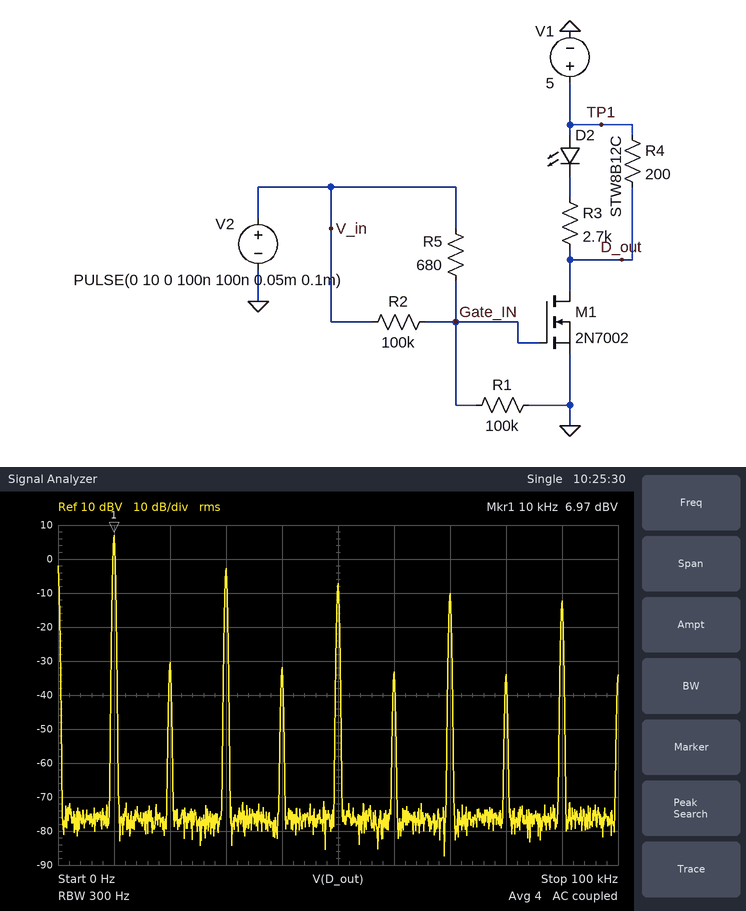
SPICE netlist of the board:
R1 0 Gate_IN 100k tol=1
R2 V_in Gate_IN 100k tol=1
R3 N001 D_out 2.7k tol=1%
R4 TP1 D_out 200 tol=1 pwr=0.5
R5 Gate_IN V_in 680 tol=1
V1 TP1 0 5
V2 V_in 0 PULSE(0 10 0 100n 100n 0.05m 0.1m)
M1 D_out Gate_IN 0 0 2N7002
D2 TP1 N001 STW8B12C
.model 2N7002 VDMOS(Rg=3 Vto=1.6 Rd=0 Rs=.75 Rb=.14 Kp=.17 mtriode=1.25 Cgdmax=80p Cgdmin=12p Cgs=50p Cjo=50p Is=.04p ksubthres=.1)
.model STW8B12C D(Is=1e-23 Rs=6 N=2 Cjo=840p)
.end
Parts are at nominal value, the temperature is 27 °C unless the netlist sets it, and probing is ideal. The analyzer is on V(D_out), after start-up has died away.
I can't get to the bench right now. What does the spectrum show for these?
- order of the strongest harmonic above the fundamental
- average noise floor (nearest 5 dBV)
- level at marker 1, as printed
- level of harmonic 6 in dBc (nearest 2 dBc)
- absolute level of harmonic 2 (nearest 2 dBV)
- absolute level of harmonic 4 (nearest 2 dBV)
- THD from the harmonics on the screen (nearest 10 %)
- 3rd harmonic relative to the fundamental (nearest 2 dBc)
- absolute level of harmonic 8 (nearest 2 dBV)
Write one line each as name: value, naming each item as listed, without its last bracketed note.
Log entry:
order of the strongest harmonic above the fundamental: 3
average noise floor: -75 dBV
level at marker 1, as printed: 6.97 dBV
level of harmonic 6 in dBc: -40 dBc
absolute level of harmonic 2: -30 dBV
absolute level of harmonic 4: -32 dBV
THD from the harmonics on the screen: 40 %
3rd harmonic relative to the fundamental: -10 dBc
absolute level of harmonic 8: -34 dBV
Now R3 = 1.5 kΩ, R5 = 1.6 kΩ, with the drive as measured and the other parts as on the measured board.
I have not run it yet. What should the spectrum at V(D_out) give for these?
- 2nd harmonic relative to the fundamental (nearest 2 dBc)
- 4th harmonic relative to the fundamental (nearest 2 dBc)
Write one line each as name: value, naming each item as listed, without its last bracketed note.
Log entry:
2nd harmonic relative to the fundamental: -34 dBc
4th harmonic relative to the fundamental: -34 dBc
